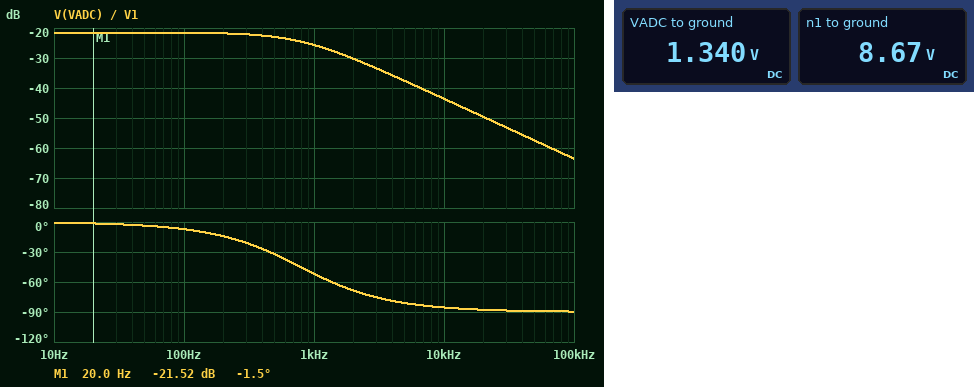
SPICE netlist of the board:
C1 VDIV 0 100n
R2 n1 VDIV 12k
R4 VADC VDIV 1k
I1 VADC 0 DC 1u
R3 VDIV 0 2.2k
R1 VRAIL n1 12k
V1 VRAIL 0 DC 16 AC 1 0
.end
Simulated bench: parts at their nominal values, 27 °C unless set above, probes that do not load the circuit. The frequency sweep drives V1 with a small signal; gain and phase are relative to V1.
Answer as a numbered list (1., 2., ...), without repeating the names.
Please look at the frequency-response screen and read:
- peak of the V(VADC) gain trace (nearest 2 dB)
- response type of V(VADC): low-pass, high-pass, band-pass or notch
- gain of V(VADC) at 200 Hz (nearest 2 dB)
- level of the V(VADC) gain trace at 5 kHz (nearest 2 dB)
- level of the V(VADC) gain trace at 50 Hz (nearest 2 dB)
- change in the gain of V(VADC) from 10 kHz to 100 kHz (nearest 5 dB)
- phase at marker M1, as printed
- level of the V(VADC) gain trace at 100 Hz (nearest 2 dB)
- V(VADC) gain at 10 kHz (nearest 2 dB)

1. -22 dB
2. low-pass
3. -22 dB
4. -38 dB
5. -22 dB
6. -20 dB
7. -1.5 deg
8. -22 dB
9. -44 dB
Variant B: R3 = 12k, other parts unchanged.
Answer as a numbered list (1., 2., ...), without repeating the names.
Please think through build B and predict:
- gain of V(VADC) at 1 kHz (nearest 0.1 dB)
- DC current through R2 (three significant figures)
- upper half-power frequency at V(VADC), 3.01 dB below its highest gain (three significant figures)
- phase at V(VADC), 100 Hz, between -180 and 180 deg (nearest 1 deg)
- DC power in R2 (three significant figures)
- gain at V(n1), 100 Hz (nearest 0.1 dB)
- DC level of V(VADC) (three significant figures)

1. -23.7 dB
2. 445 µA
3. 199 Hz
4. -27 deg
5. 2.37 mW
6. -3.9 dB
7. 5.32 V
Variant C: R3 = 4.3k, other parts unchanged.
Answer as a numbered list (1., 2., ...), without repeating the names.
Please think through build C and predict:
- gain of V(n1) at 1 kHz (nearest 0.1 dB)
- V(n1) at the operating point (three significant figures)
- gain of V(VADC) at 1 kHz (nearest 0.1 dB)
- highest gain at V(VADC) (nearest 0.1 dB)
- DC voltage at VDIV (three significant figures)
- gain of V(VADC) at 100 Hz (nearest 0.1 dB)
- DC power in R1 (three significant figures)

1. -5.8 dB
2. 9.21 V
3. -24.3 dB
4. -16.4 dB
5. 2.43 V
6. -16.6 dB
7. 3.84 mW
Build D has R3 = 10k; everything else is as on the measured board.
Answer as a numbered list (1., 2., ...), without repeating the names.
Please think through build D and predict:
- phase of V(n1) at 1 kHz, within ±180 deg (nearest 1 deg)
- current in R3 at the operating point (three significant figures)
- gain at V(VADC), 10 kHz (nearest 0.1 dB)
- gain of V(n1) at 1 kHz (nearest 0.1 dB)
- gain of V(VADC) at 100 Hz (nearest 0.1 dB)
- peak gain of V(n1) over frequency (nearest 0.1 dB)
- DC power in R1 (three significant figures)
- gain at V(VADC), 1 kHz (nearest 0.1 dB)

1. -4 deg
2. 470 µA
3. -43.6 dB
4. -5.9 dB
5. -11.4 dB
6. -3.8 dB
7. 2.66 mW
8. -23.8 dB
